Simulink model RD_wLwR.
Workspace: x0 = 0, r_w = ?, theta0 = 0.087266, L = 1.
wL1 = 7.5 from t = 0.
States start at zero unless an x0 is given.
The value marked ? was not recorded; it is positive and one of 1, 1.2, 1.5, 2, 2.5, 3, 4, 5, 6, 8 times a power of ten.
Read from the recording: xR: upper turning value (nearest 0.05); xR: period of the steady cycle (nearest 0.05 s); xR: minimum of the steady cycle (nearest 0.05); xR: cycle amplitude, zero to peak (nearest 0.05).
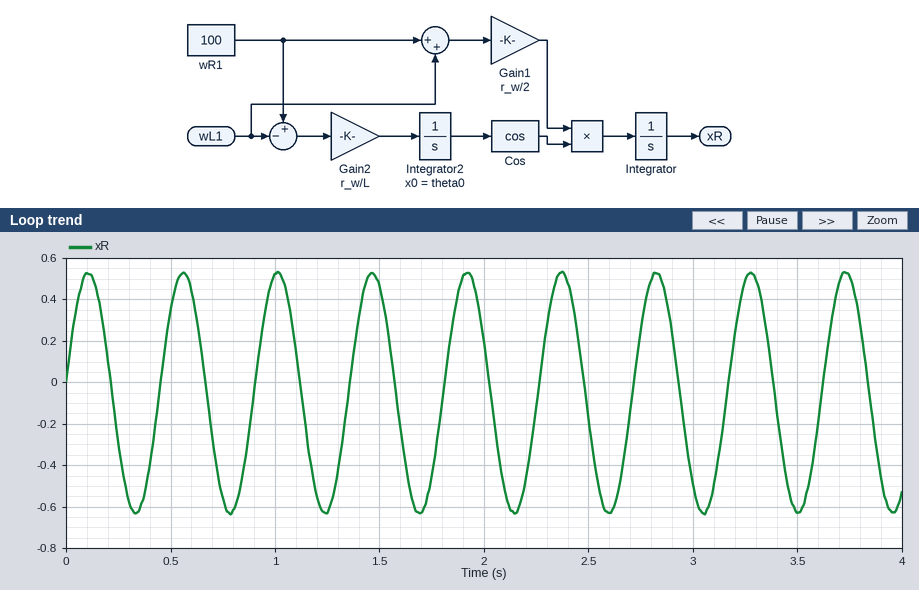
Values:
0.55
0.45 s
-0.65
0.60
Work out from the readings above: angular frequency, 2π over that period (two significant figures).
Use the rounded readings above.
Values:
14 rad/s
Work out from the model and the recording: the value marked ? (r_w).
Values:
0.15
